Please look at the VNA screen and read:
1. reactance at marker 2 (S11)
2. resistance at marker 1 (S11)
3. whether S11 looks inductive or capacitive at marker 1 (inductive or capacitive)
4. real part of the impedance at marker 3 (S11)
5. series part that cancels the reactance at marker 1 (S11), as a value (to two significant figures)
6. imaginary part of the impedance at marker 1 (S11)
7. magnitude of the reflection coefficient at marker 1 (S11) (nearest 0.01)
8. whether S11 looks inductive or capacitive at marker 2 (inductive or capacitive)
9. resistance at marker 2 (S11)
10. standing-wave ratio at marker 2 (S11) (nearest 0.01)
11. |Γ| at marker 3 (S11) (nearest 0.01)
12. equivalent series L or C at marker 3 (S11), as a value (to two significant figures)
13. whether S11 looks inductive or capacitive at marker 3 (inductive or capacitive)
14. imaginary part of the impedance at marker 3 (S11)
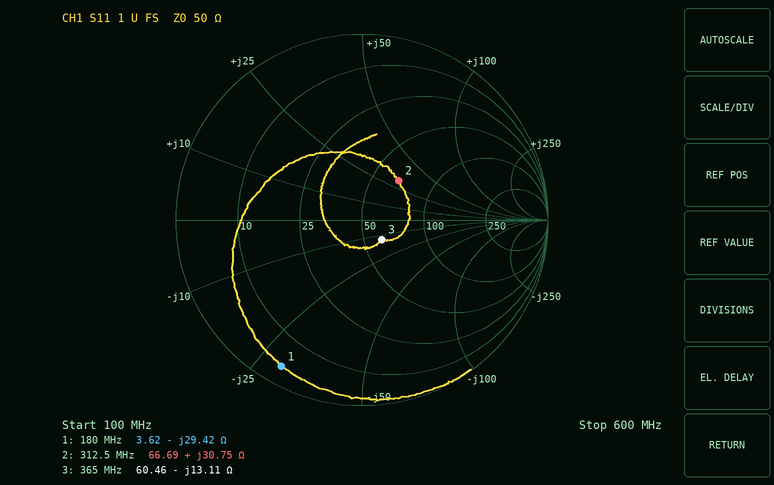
+30.75 Ω
3.62 Ω
capacitive
60.46 Ω
26 nH
-29.42 Ω
0.90
inductive
66.69 Ω
1.82
0.15
33 pF
capacitive
-13.11 Ω
